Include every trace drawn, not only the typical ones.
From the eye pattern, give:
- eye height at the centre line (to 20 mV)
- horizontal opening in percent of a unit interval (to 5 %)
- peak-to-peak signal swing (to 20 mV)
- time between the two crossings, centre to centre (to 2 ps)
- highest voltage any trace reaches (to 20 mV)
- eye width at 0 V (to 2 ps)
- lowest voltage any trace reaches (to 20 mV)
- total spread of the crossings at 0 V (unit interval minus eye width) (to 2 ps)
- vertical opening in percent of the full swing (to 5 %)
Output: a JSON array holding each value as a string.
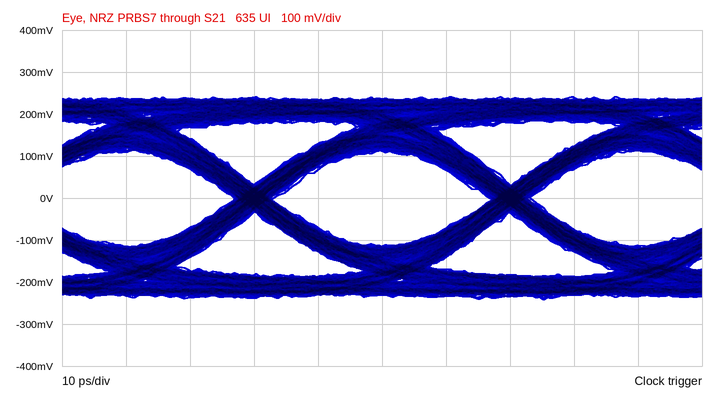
["220 mV", "85 %", "480 mV", "40 ps", "240 mV", "34 ps", "-240 mV", "6 ps", "45 %"]
